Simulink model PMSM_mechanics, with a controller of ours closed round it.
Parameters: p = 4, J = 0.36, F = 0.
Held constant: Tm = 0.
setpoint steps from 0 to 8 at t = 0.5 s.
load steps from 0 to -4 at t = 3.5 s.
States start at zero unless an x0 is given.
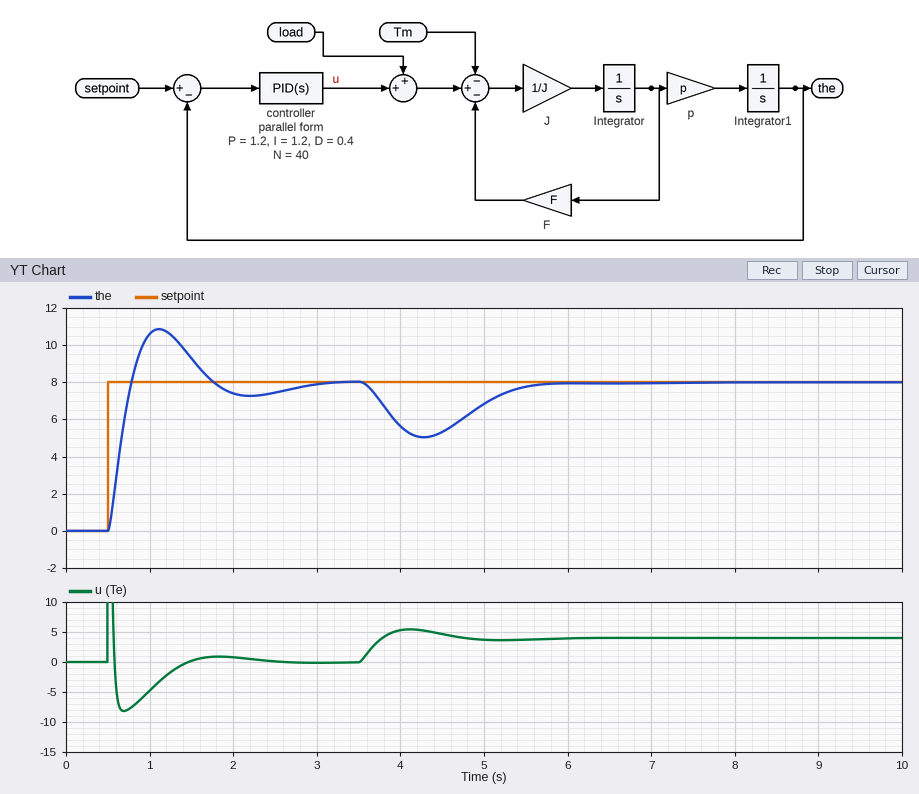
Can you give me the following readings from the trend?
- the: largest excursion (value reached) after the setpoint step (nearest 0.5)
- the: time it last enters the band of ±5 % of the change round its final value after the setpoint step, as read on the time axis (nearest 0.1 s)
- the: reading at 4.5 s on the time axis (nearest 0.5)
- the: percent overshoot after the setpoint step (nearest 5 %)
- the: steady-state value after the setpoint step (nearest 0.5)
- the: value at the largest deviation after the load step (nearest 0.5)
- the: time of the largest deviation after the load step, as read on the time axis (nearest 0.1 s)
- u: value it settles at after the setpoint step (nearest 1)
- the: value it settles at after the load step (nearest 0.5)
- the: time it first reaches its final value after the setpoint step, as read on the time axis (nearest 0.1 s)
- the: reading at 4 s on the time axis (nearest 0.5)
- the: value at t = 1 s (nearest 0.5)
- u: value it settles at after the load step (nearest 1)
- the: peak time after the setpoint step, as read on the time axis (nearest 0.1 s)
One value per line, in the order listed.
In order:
11.0
2.7 s
5.5
35 %
8.0
5.0
4.3 s
0
8.0
0.8 s
5.5
10.5
4
1.1 s
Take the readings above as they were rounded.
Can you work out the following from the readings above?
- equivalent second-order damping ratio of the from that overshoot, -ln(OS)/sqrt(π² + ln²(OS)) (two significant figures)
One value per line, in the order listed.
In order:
0.32
